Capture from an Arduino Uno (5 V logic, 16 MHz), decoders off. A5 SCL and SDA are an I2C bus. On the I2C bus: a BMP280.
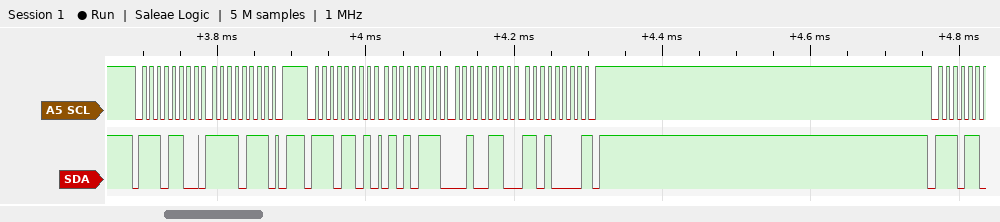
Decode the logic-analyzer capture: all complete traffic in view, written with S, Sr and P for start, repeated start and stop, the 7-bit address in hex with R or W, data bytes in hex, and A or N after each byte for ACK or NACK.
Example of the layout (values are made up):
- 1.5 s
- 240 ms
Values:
- S 76W A F7 A P S 76R A 57 A 26 A D0 N P
